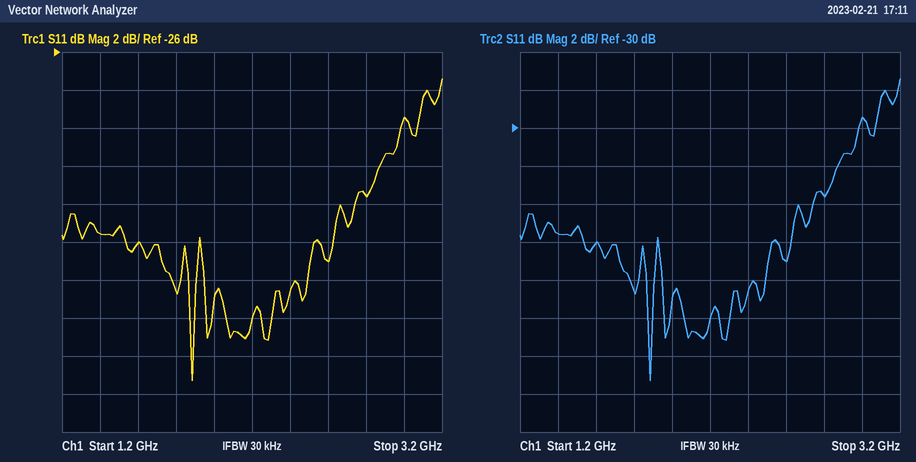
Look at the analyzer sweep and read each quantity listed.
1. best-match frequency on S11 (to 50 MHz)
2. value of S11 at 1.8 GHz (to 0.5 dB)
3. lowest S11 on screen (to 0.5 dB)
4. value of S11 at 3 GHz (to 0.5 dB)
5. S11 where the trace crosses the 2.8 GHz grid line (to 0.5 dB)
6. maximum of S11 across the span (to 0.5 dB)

1.90 GHz
-38.5 dB
-43.5 dB
-29.5 dB
-33.5 dB
-27.5 dB
